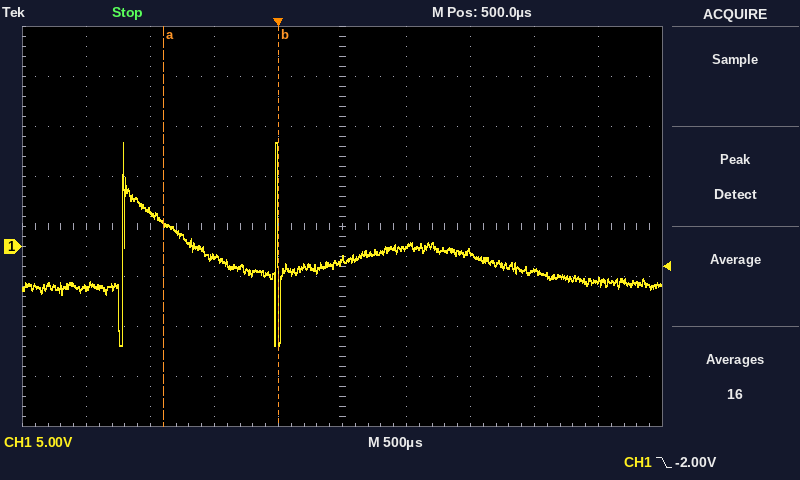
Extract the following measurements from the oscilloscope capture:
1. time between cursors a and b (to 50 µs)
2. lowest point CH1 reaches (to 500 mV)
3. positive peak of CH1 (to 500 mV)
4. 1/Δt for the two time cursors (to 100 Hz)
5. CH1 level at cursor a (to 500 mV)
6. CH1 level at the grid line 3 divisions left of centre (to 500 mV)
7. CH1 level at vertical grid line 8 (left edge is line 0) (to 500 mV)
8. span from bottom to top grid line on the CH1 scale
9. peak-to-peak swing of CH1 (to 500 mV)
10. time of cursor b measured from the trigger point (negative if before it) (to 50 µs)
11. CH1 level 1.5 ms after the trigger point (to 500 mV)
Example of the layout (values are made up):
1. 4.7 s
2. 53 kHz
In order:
1. 900 µs
2. -10.0 V
3. 10.5 V
4. 1.1 kHz
5. 2.5 V
6. 3.5 V
7. -2.5 V
8. 40 V
9. 20.5 V
10. 0 µs
11. -500 mV
